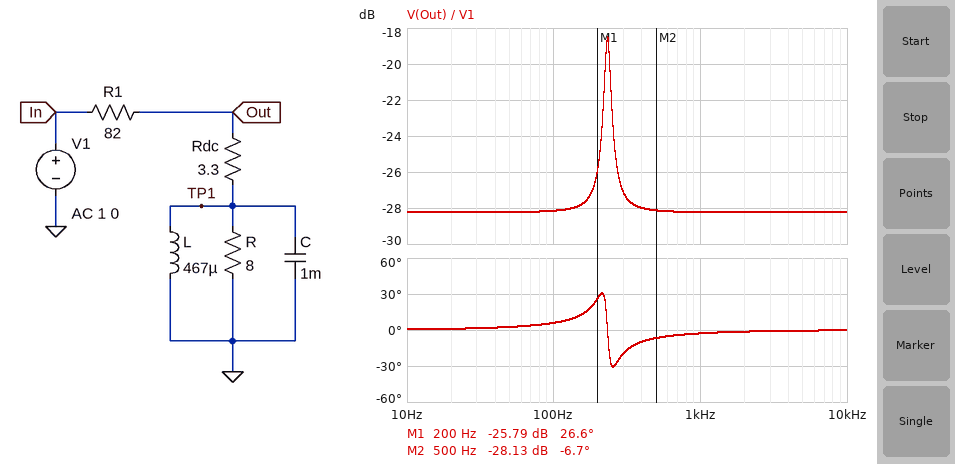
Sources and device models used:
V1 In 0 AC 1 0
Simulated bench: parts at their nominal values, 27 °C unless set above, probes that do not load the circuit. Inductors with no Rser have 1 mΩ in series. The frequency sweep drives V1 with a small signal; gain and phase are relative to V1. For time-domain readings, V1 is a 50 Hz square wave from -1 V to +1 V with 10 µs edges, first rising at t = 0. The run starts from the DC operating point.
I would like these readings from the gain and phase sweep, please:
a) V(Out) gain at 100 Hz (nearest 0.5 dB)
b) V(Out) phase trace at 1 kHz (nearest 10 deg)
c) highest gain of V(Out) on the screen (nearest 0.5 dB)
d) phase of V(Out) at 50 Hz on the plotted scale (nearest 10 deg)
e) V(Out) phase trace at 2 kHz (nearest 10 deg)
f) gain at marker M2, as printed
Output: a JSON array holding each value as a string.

["-28.0 dB", "0 deg", "-18.5 dB", "0 deg", "0 deg", "-28.13 dB"]
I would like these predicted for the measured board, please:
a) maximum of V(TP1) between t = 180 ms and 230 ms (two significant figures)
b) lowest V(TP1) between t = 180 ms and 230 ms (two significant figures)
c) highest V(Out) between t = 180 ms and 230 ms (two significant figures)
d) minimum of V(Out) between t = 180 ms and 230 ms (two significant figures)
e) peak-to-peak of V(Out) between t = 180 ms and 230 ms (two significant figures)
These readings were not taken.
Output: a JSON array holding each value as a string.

["16 mV", "-16 mV", "54 mV", "-54 mV", "110 mV"]
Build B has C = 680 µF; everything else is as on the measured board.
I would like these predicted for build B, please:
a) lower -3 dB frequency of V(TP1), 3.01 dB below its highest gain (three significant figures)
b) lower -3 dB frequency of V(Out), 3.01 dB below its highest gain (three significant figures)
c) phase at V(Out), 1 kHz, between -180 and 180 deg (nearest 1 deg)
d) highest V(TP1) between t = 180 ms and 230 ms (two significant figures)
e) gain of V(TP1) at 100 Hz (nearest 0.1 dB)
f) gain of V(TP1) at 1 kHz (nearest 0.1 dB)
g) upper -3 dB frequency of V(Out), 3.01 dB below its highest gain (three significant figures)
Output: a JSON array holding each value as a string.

["267 Hz", "265 Hz", "-4 deg", "15 mV", "-48.1 dB", "-50.5 dB", "301 Hz"]
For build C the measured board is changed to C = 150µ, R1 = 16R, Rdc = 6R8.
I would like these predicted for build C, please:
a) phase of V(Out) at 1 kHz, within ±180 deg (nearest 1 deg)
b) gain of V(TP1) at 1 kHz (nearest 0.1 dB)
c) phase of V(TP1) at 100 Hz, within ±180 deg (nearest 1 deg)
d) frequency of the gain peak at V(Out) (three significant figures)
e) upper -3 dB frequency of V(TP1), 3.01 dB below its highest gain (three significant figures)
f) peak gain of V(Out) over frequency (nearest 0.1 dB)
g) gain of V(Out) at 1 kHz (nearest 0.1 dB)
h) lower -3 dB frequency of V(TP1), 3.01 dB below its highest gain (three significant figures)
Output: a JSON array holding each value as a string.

["-9 deg", "-23.1 dB", "87 deg", "601 Hz", "698 Hz", "-6.4 dB", "-10.0 dB", "518 Hz"]
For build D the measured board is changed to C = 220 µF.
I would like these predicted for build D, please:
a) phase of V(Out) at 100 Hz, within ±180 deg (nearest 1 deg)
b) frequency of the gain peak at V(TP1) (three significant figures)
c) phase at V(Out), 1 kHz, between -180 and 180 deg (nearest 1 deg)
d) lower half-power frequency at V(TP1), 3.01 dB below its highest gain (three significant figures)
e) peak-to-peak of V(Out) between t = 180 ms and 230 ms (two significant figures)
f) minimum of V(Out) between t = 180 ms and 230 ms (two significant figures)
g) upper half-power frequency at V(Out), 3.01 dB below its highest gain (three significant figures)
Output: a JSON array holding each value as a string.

["5 deg", "497 Hz", "-15 deg", "449 Hz", "130 mV", "-66 mV", "555 Hz"]
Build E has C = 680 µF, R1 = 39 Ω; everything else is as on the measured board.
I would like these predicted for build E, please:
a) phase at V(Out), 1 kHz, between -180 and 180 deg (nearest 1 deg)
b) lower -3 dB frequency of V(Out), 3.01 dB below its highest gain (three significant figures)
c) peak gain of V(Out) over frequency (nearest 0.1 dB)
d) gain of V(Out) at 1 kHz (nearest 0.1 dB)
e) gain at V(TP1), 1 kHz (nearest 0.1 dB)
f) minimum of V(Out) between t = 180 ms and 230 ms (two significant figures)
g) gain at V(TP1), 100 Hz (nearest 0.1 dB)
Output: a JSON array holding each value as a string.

["-4 deg", "263 Hz", "-13.0 dB", "-22.1 dB", "-44.4 dB", "-110 mV", "-42.0 dB"]
